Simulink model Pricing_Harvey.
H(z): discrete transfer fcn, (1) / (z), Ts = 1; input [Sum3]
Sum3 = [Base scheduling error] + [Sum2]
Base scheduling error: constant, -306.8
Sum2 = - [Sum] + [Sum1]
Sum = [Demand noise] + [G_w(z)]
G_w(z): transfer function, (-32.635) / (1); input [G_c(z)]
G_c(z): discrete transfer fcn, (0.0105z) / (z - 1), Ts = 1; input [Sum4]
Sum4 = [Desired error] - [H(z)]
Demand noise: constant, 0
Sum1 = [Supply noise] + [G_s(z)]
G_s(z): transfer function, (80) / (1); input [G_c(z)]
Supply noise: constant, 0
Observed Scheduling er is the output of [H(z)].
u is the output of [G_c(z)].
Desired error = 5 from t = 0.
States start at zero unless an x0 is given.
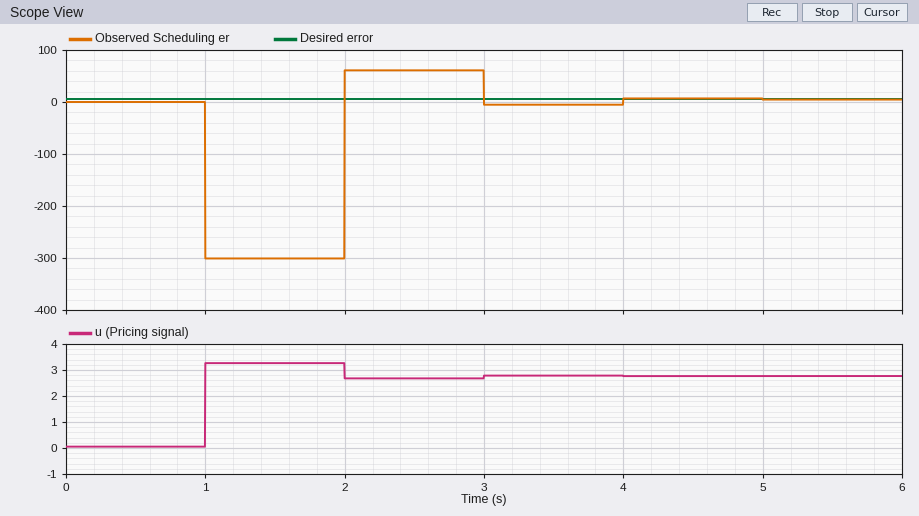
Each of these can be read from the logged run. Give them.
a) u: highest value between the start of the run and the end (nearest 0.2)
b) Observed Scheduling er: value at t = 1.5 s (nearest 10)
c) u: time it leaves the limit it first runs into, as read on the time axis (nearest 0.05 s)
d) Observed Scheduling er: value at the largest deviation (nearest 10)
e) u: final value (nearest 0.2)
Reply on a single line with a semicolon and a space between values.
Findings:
3.2; -300; 1.00 s; -300; 2.8
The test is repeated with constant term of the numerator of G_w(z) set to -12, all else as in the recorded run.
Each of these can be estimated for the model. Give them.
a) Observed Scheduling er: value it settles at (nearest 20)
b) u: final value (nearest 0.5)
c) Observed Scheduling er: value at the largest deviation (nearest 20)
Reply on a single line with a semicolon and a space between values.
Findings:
0; 3.5; -300
